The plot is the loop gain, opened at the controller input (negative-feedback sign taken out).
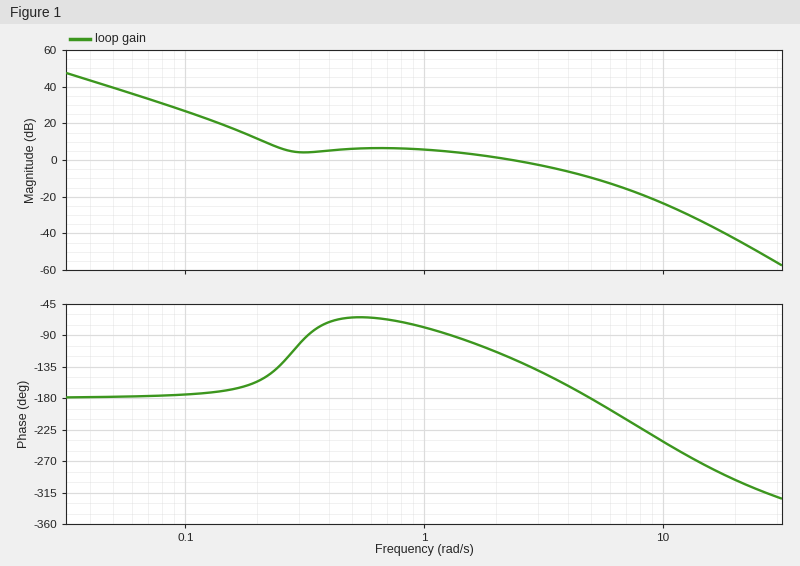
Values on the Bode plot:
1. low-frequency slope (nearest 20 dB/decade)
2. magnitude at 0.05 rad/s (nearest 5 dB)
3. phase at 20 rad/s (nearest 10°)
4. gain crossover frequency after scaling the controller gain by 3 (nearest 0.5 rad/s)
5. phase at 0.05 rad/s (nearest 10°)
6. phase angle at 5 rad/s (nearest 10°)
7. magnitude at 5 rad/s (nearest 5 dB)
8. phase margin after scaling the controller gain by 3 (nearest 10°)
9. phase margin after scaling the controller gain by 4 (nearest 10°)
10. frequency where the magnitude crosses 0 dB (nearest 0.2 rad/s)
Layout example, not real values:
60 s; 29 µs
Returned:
-40 dB/decade; 40 dB; -300°; 5.0 rad/s; -180°; -180°; -10 dB; 0°; -10°; 2.4 rad/s
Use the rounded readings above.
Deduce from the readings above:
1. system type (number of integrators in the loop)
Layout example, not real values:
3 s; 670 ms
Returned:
2
